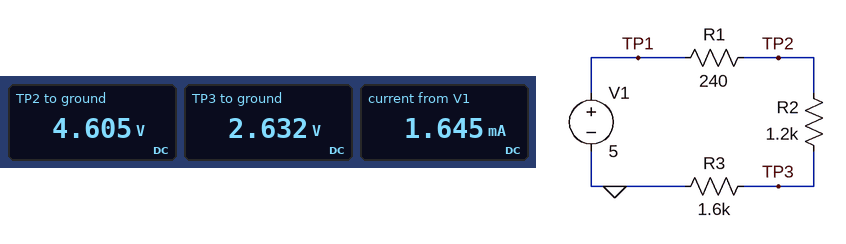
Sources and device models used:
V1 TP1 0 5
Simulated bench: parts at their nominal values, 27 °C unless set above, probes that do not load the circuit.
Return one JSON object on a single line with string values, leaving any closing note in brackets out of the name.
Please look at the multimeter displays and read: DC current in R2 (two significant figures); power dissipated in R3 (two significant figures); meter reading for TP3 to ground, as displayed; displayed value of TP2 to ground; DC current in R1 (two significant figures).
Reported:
{"DC current in R2": "1.6 mA", "power dissipated in R3": "4.3 mW", "meter reading for TP3 to ground, as displayed": "2.632 V", "displayed value of TP2 to ground": "4.605 V", "DC current in R1": "1.6 mA"}
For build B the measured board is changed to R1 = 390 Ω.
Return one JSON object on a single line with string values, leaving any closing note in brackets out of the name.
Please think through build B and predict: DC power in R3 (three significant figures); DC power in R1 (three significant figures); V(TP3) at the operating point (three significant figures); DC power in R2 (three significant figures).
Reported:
{"DC power in R3": "3.93 mW", "DC power in R1": "958 µW", "V(TP3) at the operating point": "2.51 V", "DC power in R2": "2.95 mW"}
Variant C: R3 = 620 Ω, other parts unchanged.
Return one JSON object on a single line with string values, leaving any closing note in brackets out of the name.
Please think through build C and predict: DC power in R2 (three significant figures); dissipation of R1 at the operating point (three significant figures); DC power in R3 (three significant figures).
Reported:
{"DC power in R2": "7.07 mW", "dissipation of R1 at the operating point": "1.41 mW", "DC power in R3": "3.65 mW"}
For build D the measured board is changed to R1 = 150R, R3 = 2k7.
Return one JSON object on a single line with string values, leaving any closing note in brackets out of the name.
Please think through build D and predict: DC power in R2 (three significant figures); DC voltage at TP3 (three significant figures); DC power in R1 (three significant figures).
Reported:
{"DC power in R2": "1.83 mW", "DC voltage at TP3": "3.33 V", "DC power in R1": "229 µW"}
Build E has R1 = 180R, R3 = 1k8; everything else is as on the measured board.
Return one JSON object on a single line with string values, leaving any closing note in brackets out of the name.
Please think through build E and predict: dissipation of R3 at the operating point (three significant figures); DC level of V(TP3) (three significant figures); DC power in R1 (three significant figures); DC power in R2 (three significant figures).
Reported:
{"dissipation of R3 at the operating point": "4.45 mW", "DC level of V(TP3)": "2.83 V", "DC power in R1": "445 µW", "DC power in R2": "2.97 mW"}
